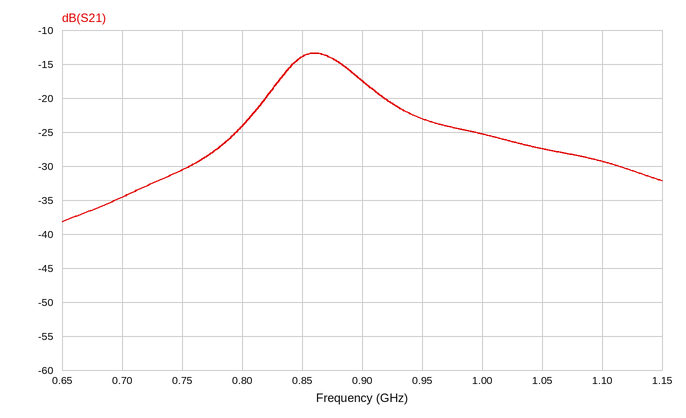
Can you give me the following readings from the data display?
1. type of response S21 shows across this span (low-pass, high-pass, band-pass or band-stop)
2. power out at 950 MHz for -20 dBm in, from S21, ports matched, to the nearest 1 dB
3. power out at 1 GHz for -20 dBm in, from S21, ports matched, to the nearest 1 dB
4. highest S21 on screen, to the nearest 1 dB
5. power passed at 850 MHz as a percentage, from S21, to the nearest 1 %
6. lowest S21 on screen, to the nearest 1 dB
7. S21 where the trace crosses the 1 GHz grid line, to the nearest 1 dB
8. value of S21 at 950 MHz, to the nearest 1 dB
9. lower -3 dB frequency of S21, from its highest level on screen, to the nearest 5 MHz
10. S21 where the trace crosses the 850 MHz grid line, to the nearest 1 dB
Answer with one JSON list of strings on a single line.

["band-pass", "-43 dBm", "-45 dBm", "-13 dB", "4 %", "-38 dB", "-25 dB", "-23 dB", "835 MHz", "-14 dB"]
